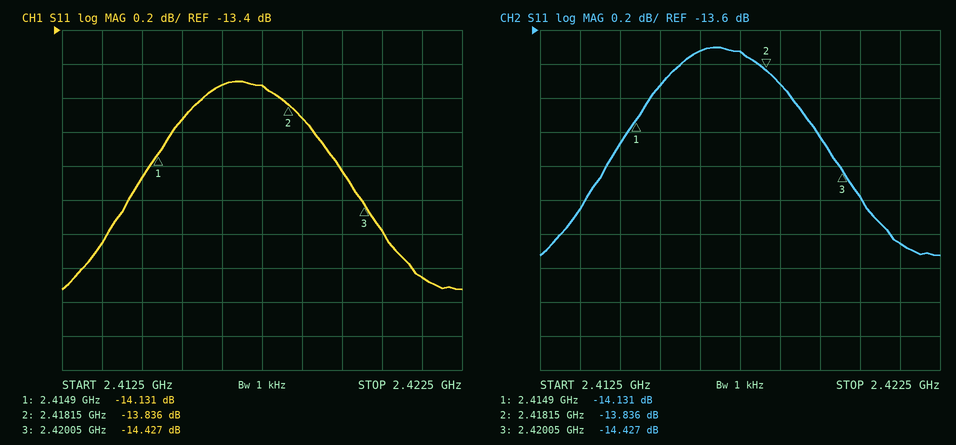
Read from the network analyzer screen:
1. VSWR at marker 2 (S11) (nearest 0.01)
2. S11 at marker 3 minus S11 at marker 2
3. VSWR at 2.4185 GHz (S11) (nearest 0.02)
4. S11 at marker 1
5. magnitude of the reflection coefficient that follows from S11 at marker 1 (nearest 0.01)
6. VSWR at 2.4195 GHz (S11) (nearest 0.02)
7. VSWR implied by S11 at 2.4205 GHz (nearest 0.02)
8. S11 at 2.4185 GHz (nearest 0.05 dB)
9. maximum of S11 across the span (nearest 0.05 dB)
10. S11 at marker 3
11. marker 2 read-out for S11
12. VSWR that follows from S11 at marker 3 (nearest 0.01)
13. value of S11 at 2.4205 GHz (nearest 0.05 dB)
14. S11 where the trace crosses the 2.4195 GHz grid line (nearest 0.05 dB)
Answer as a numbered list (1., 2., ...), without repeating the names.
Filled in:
1. 1.51
2. -0.591 dB
3. 1.50
4. -14.131 dB
5. 0.20
6. 1.48
7. 1.46
8. -13.90 dB
9. -13.70 dB
10. -14.427 dB
11. -13.836 dB
12. 1.47
13. -14.60 dB
14. -14.25 dB
